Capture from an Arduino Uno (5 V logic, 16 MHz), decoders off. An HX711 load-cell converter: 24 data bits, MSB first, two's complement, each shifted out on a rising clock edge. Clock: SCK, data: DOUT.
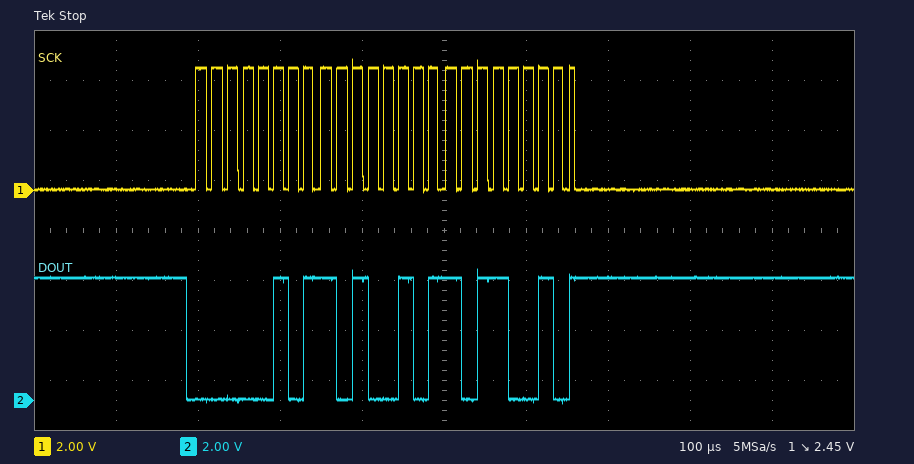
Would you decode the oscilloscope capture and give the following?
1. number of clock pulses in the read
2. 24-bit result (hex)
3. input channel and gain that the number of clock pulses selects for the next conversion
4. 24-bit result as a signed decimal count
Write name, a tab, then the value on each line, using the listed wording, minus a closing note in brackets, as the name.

number of clock pulses in the read	25
24-bit result	0x05A5B2
input channel and gain that the number of clock pulses selects for the next conversion	channel A, gain 128
24-bit result as a signed decimal count	370098
